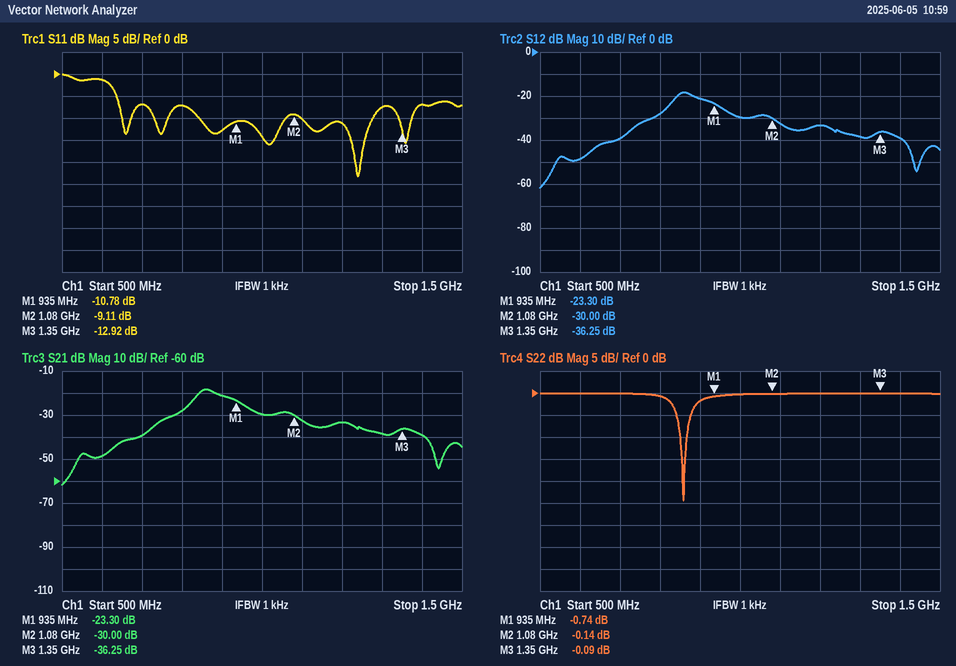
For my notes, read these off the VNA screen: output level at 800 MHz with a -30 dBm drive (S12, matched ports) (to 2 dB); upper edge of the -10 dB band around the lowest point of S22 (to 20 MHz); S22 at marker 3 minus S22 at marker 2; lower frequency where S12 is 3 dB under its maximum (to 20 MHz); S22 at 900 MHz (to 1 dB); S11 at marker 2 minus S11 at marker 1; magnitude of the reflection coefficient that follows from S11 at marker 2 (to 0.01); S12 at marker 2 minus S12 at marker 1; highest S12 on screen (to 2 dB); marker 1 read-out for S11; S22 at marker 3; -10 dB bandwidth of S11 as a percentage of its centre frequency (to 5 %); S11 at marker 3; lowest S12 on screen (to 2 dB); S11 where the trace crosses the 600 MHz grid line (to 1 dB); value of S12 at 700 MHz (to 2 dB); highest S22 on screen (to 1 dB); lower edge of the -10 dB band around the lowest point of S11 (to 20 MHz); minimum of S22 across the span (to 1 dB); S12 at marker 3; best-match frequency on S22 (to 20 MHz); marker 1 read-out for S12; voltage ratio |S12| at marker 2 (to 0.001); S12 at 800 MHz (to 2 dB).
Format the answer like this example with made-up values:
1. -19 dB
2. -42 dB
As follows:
1. -58 dBm
2. 860 MHz
3. 0.05 dB
4. 840 MHz
5. -2 dB
6. 1.67 dB
7. 0.35
8. -6.70 dB
9. -18 dB
10. -10.78 dB
11. -0.09 dB
12. 15 %
13. -12.92 dB
14. -62 dB
15. -1 dB
16. -40 dB
17. 0 dB
18. 1.10 GHz
19. -24 dB
20. -36.25 dB
21. 860 MHz
22. -23.30 dB
23. 0.032
24. -28 dB
